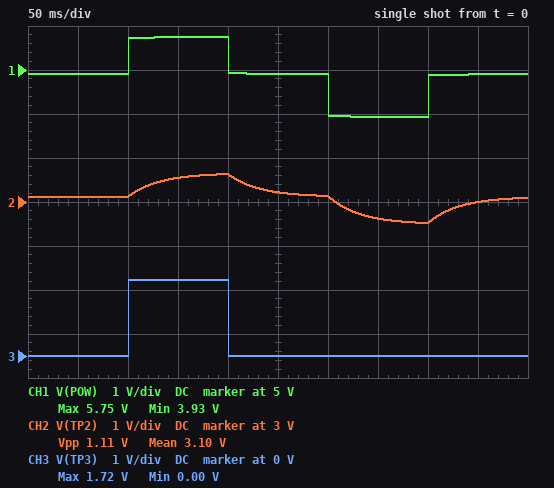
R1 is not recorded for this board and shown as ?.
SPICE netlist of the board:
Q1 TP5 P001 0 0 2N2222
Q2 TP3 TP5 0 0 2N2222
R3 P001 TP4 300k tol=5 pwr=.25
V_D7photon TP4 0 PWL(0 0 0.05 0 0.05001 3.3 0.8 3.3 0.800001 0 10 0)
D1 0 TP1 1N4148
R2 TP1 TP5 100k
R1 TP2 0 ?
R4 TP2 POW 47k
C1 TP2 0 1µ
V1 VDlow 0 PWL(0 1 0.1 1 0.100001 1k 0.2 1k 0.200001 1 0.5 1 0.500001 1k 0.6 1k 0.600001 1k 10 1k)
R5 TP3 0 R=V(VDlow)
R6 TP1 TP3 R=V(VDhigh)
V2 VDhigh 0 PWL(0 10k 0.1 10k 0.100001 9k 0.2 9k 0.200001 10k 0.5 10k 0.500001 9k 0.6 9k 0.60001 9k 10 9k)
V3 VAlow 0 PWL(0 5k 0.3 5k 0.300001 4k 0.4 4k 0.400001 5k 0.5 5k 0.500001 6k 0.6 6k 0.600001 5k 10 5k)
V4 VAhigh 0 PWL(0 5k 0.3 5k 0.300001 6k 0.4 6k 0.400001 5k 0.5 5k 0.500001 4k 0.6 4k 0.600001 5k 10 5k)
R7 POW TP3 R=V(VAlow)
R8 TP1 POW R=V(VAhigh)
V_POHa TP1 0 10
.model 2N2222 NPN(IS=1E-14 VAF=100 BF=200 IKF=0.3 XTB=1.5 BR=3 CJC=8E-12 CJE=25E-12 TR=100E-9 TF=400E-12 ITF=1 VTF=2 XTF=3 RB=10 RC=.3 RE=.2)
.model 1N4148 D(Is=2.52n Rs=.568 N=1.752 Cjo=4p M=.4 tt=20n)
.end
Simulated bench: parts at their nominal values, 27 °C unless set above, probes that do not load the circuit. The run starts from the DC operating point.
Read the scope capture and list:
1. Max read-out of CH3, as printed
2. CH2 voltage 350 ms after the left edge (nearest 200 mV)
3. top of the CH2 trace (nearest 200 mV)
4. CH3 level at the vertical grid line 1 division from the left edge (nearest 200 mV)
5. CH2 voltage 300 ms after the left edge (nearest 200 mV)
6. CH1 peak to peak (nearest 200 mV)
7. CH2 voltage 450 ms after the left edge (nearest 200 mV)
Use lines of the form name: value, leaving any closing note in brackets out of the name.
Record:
Max read-out of CH3, as printed: 1.72 V
CH2 voltage 350 ms after the left edge: 2.6 V
top of the CH2 trace: 3.6 V
CH3 level at the vertical grid line 1 division from the left edge: 0 V
CH2 voltage 300 ms after the left edge: 3.2 V
CH1 peak to peak: 1.8 V
CH2 voltage 450 ms after the left edge: 3.0 V
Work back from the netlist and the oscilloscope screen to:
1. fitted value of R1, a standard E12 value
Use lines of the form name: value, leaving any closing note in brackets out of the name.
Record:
fitted value of R1, a standard E12 value: 82 kΩ
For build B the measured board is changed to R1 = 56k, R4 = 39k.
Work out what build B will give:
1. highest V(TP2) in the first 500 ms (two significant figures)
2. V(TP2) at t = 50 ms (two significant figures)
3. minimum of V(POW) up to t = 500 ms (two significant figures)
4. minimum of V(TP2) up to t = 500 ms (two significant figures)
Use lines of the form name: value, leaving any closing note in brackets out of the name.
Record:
highest V(TP2) in the first 500 ms: 3.4 V
V(TP2) at t = 50 ms: 2.9 V
minimum of V(POW) up to t = 500 ms: 3.9 V
minimum of V(TP2) up to t = 500 ms: 2.3 V
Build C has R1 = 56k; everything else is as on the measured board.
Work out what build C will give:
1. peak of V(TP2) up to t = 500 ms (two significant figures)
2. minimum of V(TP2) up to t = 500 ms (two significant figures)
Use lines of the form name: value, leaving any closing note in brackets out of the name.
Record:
peak of V(TP2) up to t = 500 ms: 3.1 V
minimum of V(TP2) up to t = 500 ms: 2.1 V
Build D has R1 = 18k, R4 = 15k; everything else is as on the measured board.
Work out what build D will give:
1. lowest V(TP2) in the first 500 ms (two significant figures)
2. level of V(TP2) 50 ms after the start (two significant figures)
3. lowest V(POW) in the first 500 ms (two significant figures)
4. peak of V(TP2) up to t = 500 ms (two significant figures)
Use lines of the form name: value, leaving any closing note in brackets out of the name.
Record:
lowest V(TP2) in the first 500 ms: 2.0 V
level of V(TP2) 50 ms after the start: 2.5 V
lowest V(POW) in the first 500 ms: 3.7 V
peak of V(TP2) up to t = 500 ms: 3.0 V
